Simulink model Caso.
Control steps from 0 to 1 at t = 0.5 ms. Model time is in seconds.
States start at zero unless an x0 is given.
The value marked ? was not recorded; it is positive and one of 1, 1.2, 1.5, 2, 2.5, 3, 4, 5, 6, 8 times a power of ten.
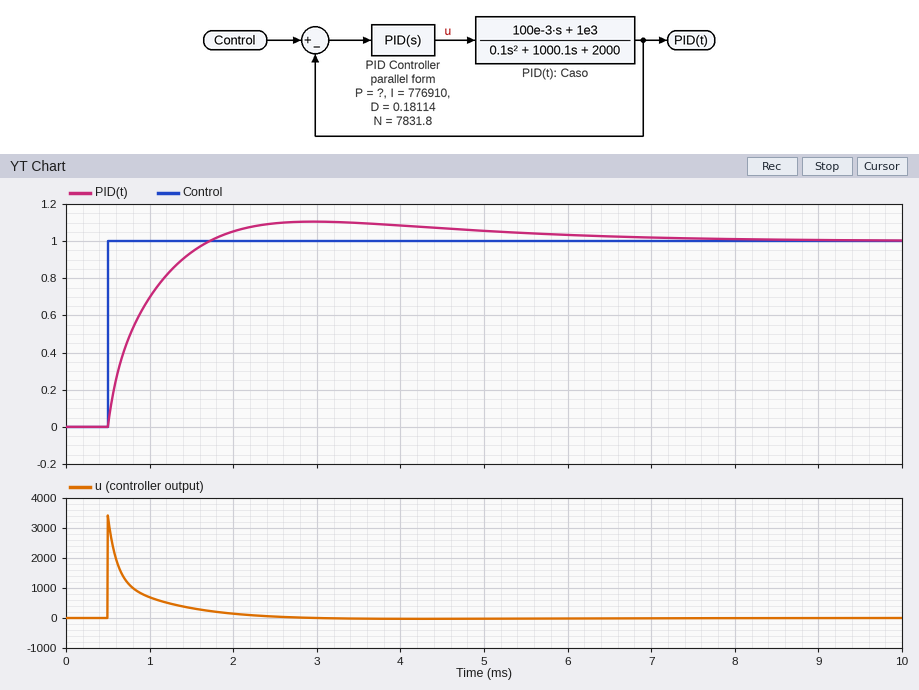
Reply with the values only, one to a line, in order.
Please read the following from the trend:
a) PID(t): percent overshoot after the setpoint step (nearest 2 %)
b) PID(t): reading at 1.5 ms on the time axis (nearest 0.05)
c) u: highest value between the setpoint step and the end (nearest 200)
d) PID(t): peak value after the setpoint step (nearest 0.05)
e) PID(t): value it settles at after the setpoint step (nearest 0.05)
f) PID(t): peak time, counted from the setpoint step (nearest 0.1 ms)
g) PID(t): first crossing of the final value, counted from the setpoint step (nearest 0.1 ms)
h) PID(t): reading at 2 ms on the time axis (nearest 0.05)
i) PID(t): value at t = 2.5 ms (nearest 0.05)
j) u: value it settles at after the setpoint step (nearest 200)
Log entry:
10 %
0.95
3400
1.10
1.00
2.5 ms
1.2 ms
1.05
1.10
0
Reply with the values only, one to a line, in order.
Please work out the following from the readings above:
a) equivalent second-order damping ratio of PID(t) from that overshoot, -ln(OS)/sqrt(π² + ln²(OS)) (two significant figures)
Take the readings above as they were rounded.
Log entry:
0.59
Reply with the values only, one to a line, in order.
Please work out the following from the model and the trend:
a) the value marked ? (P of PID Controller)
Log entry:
2000
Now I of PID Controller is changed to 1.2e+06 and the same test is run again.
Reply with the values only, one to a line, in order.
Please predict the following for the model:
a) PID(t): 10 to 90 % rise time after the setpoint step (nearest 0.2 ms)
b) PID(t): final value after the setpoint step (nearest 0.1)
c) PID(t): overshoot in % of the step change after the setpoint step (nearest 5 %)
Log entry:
0.8 ms
1.0
15 %
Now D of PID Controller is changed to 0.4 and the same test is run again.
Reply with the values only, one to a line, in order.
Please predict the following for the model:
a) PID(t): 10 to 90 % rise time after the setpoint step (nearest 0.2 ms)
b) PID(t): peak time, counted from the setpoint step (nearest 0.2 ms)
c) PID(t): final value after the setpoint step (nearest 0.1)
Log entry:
1.0 ms
2.8 ms
1.0
